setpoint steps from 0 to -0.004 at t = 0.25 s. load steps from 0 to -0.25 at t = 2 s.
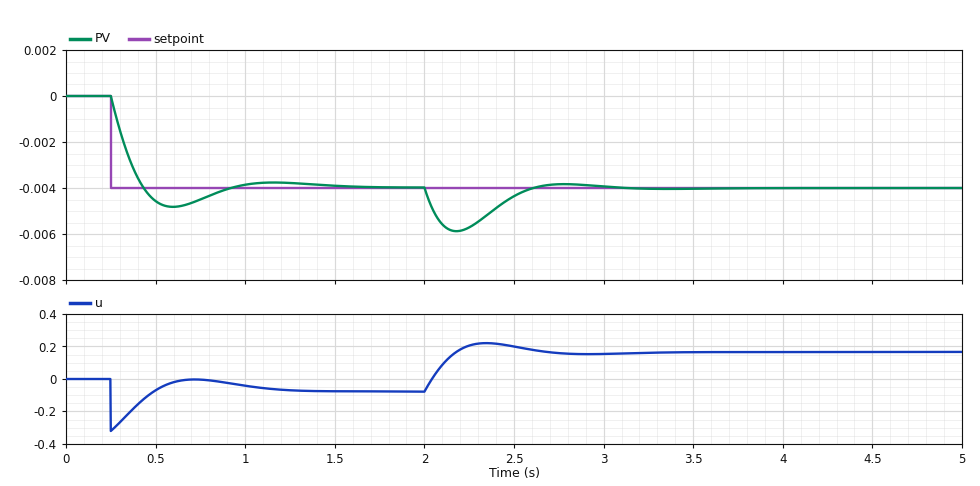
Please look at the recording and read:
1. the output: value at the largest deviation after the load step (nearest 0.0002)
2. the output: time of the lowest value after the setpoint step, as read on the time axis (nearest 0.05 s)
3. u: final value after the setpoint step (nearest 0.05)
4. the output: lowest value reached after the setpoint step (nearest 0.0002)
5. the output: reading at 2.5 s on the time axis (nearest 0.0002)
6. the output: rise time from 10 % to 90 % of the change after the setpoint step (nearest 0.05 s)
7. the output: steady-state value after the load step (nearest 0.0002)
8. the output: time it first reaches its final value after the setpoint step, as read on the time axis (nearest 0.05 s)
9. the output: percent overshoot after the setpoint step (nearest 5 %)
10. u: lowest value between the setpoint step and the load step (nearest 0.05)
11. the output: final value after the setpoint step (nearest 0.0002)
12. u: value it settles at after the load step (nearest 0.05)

-0.0058
0.60 s
-0.10
-0.0048
-0.0044
0.15 s
-0.0040
0.45 s
20 %
-0.30
-0.0040
0.15
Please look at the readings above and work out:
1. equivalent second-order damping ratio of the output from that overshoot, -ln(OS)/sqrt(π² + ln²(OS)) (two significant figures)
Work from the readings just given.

0.46
